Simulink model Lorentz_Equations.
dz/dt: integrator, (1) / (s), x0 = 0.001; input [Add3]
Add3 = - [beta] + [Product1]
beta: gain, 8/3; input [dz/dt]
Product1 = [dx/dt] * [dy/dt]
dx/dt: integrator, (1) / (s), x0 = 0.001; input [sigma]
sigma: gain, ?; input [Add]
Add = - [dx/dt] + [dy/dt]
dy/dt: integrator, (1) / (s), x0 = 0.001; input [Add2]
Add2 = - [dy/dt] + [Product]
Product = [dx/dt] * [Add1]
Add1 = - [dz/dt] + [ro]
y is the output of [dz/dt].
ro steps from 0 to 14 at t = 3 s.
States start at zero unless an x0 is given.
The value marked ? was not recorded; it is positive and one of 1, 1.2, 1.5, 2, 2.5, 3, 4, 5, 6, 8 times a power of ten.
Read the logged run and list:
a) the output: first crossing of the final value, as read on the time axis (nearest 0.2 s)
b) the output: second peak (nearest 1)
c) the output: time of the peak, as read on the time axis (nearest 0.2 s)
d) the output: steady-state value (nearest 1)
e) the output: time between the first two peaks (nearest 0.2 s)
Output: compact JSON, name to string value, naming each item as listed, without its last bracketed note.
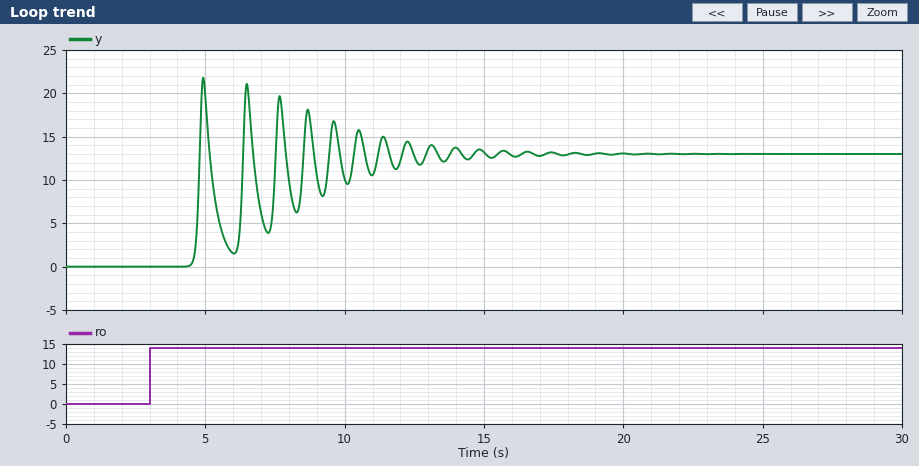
{"the output: first crossing of the final value, as read on the time axis": "4.8 s", "the output: second peak": "21", "the output: time of the peak, as read on the time axis": "5.0 s", "the output: steady-state value": "13", "the output: time between the first two peaks": "1.6 s"}
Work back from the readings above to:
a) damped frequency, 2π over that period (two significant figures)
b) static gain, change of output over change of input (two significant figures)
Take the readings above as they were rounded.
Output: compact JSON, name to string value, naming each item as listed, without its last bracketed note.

{"damped frequency, 2π over that period": "3.9 rad/s", "static gain, change of output over change of input": "0.93"}
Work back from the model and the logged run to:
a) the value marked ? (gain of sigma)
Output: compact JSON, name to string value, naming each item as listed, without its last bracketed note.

{"the value marked ?": "10"}
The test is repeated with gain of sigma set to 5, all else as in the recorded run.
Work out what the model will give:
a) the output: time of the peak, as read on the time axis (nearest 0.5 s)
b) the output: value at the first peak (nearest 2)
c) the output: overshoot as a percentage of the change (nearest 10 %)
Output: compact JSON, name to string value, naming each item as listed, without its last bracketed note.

{"the output: time of the peak, as read on the time axis": "5.5 s", "the output: value at the first peak": "22", "the output: overshoot as a percentage of the change": "60 %"}
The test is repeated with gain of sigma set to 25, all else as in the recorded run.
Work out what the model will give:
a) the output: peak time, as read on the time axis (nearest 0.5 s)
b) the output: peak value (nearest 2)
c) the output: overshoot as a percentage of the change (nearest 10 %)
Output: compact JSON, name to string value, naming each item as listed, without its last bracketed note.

{"the output: peak time, as read on the time axis": "4.5 s", "the output: peak value": "22", "the output: overshoot as a percentage of the change": "70 %"}
